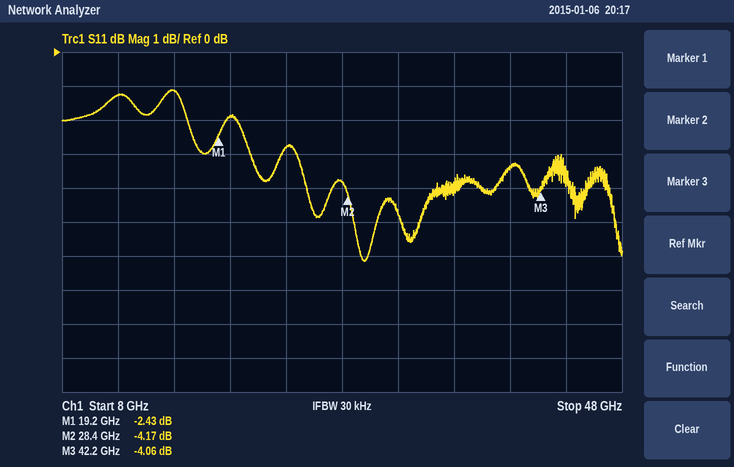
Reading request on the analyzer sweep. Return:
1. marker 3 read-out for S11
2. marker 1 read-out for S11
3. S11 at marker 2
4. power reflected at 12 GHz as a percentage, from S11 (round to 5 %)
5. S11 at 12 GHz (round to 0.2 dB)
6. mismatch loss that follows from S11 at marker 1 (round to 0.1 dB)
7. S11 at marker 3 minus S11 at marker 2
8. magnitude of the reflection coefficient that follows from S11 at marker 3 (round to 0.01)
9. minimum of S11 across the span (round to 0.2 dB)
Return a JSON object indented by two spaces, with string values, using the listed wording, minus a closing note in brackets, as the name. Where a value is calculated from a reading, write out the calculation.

{
  "marker 3 read-out for S11": "-4.06 dB",
  "marker 1 read-out for S11": "-2.43 dB",
  "S11 at marker 2": "-4.17 dB",
  "power reflected at 12 GHz as a percentage, from S11": "10^(-1.2/10) ≈ 75.9 %, so 75 % to the nearest 5 %",
  "S11 at 12 GHz": "-1.2 dB",
  "mismatch loss that follows from S11 at marker 1": "−10 log10(1 − 10^(-2.43/10)) ≈ 3.7 dB",
  "S11 at marker 3 minus S11 at marker 2": "-4.06 − (-4.17) = 0.11 dB",
  "magnitude of the reflection coefficient that follows from S11 at marker 3": "10^(-4.06/20) ≈ 0.63",
  "minimum of S11 across the span": "-6.2 dB"
}
